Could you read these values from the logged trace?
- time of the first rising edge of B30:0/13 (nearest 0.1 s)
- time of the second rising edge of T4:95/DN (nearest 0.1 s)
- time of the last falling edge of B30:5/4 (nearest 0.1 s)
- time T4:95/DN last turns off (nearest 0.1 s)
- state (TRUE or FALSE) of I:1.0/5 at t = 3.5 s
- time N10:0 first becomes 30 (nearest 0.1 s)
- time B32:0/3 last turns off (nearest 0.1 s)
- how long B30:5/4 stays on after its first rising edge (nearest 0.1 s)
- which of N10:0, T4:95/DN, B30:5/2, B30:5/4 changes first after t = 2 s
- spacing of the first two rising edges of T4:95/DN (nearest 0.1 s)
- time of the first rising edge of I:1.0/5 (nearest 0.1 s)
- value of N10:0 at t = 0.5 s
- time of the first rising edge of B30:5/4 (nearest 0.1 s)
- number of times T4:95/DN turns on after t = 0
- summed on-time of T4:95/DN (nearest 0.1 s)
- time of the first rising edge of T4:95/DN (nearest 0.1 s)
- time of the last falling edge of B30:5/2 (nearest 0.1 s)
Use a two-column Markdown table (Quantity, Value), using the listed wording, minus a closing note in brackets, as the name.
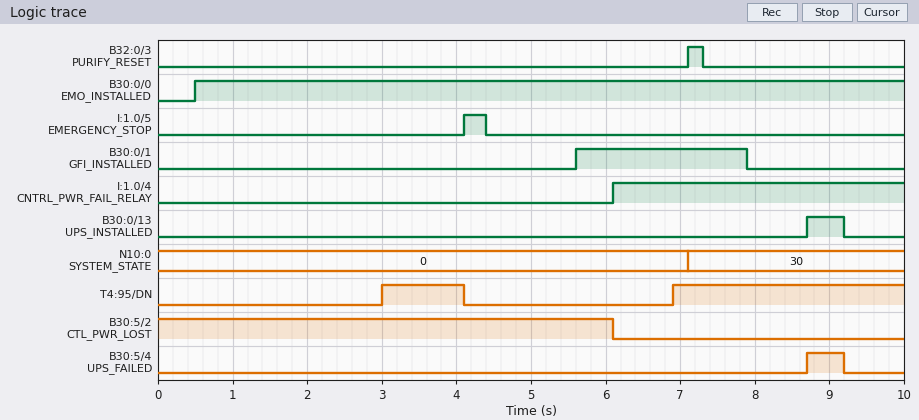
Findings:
| Quantity | Value |
|---|---|
| time of the first rising edge of B30:0/13 | 8.7 s |
| time of the second rising edge of T4:95/DN | 6.9 s |
| time of the last falling edge of B30:5/4 | 9.2 s |
| time T4:95/DN last turns off | 4.1 s |
| state (TRUE or FALSE) of I:1.0/5 at t = 3.5 s | FALSE |
| time N10:0 first becomes 30 | 7.1 s |
| time B32:0/3 last turns off | 7.3 s |
| how long B30:5/4 stays on after its first rising edge | 0.5 s |
| which of N10:0, T4:95/DN, B30:5/2, B30:5/4 changes first after t = 2 s | T4:95/DN |
| spacing of the first two rising edges of T4:95/DN | 3.9 s |
| time of the first rising edge of I:1.0/5 | 4.1 s |
| value of N10:0 at t = 0.5 s | 0 |
| time of the first rising edge of B30:5/4 | 8.7 s |
| number of times T4:95/DN turns on after t = 0 | 2 |
| summed on-time of T4:95/DN | 4.2 s |
| time of the first rising edge of T4:95/DN | 3.0 s |
| time of the last falling edge of B30:5/2 | 6.1 s |
